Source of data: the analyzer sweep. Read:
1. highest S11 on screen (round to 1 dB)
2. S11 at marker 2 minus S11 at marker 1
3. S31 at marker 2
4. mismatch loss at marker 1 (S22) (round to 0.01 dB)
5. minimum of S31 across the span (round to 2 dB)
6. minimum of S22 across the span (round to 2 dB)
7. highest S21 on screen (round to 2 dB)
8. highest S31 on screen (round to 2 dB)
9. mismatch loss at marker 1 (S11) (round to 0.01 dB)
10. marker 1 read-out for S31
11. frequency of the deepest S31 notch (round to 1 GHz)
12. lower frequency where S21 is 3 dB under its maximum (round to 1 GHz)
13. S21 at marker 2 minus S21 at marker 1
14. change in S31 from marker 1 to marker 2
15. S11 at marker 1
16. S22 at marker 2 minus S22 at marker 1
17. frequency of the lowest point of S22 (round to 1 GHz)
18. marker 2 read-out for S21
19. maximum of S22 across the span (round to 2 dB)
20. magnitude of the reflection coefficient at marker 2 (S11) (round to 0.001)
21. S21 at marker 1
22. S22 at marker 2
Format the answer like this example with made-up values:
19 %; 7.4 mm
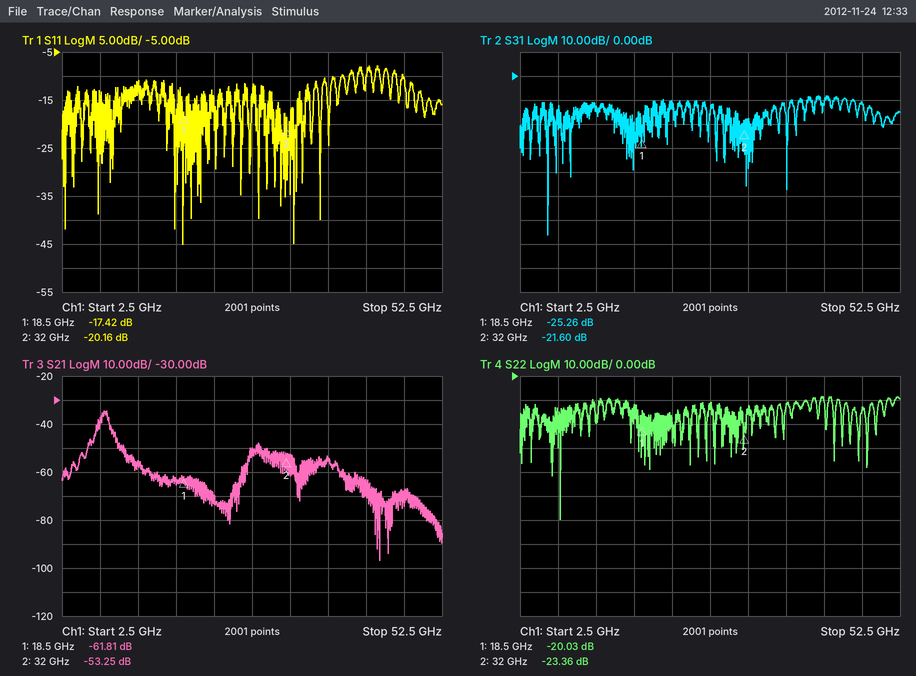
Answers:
-8 dB; -2.74 dB; -21.60 dB; 0.04 dB; -66 dB; -60 dB; -34 dB; -8 dB; 0.08 dB; -25.26 dB; 6 GHz; 8 GHz; 8.56 dB; 3.66 dB; -17.42 dB; -3.33 dB; 8 GHz; -53.25 dB; -8 dB; 0.098; -61.81 dB; -23.36 dB
